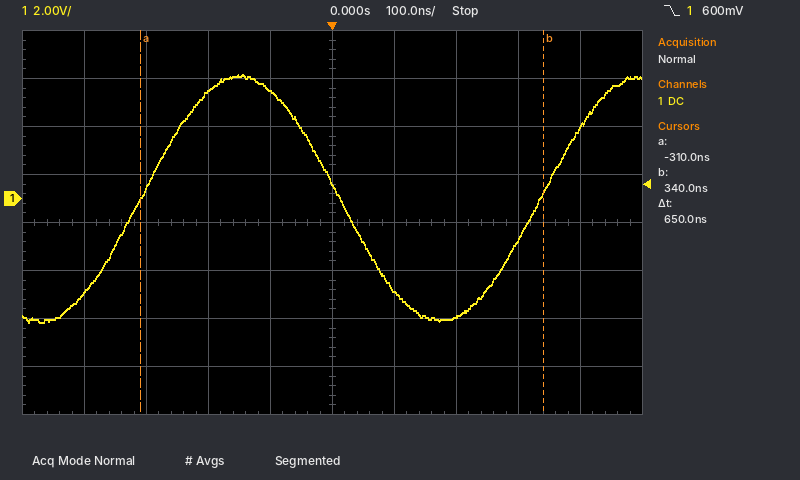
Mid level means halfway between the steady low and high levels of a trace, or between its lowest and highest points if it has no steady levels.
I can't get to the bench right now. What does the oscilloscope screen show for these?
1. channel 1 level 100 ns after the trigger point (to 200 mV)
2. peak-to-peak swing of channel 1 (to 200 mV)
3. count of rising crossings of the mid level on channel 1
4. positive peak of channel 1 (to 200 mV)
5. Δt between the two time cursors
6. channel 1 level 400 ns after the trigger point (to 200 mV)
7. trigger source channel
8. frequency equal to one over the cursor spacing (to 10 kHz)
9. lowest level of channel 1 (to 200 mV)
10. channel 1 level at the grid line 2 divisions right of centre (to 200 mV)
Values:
-3.8 V
10.4 V
2
5.2 V
650 ns
3.0 V
channel 1
1.54 MHz
-5.2 V
-5.0 V
